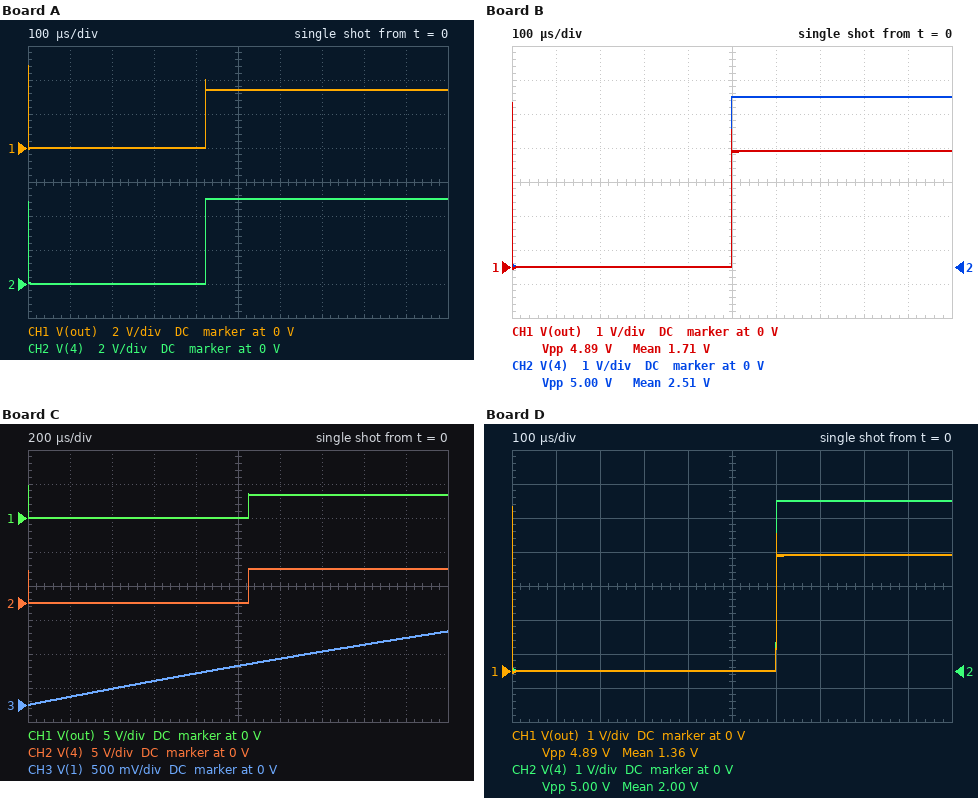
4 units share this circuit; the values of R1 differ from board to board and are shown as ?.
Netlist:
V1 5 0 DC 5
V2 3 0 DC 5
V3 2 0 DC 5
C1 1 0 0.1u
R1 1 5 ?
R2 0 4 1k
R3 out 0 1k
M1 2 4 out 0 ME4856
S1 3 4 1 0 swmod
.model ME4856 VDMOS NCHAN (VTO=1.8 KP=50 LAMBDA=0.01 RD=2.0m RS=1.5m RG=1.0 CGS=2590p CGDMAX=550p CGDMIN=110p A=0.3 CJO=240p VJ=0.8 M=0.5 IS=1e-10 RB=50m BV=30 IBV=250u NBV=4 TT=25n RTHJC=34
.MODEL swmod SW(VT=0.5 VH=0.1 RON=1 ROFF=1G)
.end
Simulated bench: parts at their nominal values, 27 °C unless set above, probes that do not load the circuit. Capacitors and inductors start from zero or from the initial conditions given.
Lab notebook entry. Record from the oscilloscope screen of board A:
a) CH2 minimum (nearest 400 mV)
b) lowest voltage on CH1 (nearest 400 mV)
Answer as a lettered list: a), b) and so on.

a) 0 V
b) 0 V
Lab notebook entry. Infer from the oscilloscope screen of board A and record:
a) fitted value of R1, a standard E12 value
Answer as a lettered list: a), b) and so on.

a) 33 kΩ
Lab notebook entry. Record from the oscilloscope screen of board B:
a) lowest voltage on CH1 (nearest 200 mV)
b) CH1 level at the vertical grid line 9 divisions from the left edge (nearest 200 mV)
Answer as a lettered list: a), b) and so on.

a) 0 V
b) 3.4 V
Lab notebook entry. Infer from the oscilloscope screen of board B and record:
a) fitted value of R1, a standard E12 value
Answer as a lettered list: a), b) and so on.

a) 39 kΩ
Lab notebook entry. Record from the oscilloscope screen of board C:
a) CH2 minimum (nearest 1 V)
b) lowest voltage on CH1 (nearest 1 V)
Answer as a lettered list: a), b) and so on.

a) 0 V
b) 0 V
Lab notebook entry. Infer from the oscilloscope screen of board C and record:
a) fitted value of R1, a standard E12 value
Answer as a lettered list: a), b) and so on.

a) 82 kΩ
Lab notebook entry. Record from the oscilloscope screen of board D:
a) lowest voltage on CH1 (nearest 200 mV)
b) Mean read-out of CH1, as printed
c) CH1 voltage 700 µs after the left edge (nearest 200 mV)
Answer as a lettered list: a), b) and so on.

a) 0 V
b) 1.36 V
c) 3.4 V
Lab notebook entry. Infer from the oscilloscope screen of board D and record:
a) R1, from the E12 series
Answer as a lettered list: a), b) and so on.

a) 47 kΩ
